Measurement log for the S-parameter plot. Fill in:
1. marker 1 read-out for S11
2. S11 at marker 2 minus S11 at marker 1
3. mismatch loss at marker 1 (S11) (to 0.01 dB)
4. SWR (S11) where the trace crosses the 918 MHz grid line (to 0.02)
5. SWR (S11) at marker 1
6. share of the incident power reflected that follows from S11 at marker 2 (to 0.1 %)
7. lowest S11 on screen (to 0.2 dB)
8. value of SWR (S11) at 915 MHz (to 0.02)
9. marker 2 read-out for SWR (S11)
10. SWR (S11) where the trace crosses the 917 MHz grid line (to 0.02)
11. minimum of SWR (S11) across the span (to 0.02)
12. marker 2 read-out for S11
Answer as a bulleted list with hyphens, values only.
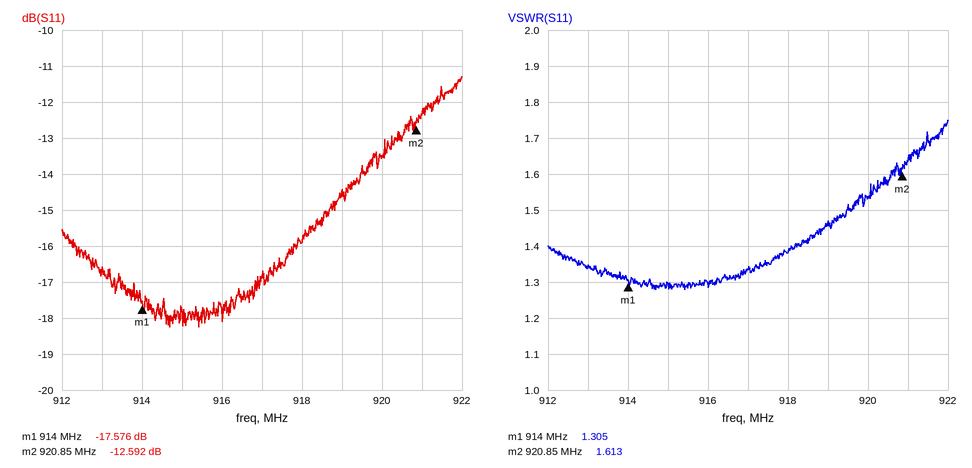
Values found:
- -17.576 dB
- 4.984 dB
- 0.08 dB
- 1.38
- 1.305
- 5.5 %
- -18.2 dB
- 1.30
- 1.613
- 1.34
- 1.28
- -12.592 dB
